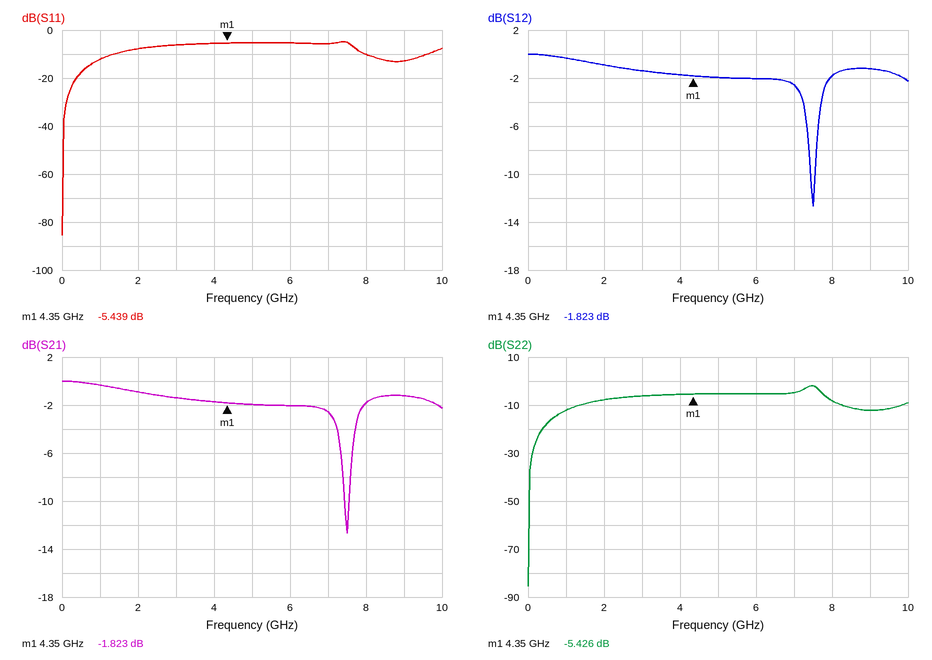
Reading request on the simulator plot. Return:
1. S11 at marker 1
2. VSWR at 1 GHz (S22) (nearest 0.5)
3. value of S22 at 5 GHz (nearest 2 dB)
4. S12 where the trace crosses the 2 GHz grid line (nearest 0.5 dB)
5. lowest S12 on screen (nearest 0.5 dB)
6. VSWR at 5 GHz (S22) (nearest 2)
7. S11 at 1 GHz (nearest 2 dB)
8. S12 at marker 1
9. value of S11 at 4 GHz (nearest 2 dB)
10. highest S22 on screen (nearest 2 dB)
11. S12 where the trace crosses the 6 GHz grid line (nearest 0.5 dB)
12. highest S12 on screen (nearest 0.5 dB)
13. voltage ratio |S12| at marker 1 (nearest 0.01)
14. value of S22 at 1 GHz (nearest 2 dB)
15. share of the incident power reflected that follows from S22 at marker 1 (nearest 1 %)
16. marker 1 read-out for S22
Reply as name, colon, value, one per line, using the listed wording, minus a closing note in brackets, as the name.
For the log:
S11 at marker 1: -5.439 dB
VSWR at 1 GHz (S22): 1.5
value of S22 at 5 GHz: -6 dB
S12 where the trace crosses the 2 GHz grid line: -1.0 dB
lowest S12 on screen: -12.5 dB
VSWR at 5 GHz (S22): 4
S11 at 1 GHz: -12 dB
S12 at marker 1: -1.823 dB
value of S11 at 4 GHz: -6 dB
highest S22 on screen: -2 dB
S12 where the trace crosses the 6 GHz grid line: -2.0 dB
highest S12 on screen: 0.0 dB
voltage ratio |S12| at marker 1: 0.81
value of S22 at 1 GHz: -12 dB
share of the incident power reflected that follows from S22 at marker 1: 29 %
marker 1 read-out for S22: -5.426 dB
